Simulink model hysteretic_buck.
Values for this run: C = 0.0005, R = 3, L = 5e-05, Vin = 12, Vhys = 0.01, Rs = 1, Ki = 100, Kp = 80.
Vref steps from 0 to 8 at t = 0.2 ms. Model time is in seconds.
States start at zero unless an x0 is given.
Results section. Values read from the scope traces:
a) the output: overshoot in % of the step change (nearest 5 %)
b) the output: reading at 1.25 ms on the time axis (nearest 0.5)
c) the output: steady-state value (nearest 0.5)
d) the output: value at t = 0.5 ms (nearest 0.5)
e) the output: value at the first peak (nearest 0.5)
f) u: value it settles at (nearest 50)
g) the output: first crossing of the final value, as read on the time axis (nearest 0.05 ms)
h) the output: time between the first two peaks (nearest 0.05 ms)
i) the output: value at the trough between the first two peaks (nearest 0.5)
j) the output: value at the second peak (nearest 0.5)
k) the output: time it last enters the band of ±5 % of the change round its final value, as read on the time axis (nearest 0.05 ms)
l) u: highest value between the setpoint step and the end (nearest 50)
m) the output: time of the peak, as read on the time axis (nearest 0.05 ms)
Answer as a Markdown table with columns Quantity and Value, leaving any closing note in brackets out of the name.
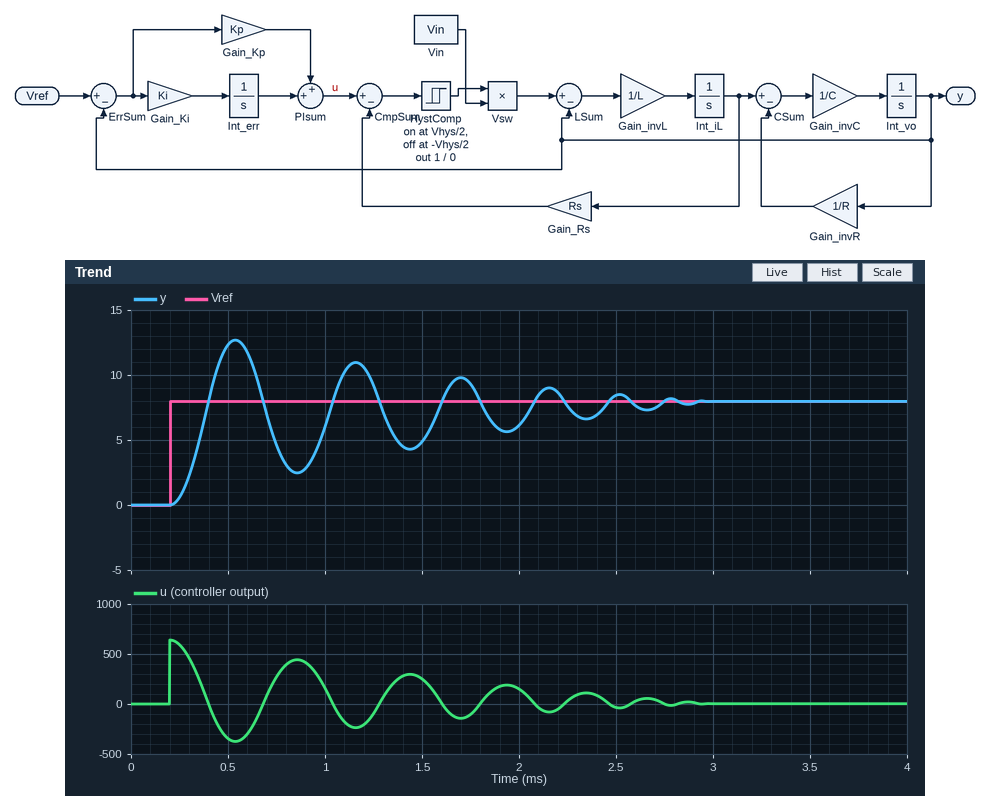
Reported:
| Quantity | Value |
|---|---|
| the output: overshoot in % of the step change | 60 % |
| the output: reading at 1.25 ms on the time axis | 9.0 |
| the output: steady-state value | 8.0 |
| the output: value at t = 0.5 ms | 12.5 |
| the output: value at the first peak | 12.5 |
| u: value it settles at | 0 |
| the output: first crossing of the final value, as read on the time axis | 0.40 ms |
| the output: time between the first two peaks | 0.60 ms |
| the output: value at the trough between the first two peaks | 2.5 |
| the output: value at the second peak | 11.0 |
| the output: time it last enters the band of ±5 % of the change round its final value, as read on the time axis | 2.70 ms |
| u: highest value between the setpoint step and the end | 650 |
| the output: time of the peak, as read on the time axis | 0.55 ms |
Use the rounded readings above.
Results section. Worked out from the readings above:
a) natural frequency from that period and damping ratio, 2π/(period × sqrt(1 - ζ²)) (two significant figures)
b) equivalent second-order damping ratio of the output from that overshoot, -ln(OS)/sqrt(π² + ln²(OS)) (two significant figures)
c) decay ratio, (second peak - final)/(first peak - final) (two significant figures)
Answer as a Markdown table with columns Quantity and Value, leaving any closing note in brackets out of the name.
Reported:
| Quantity | Value |
|---|---|
| natural frequency from that period and damping ratio, 2π/(period × sqrt(1 - ζ²)) | 11 rad/ms |
| equivalent second-order damping ratio of the output from that overshoot, -ln(OS)/sqrt(π² + ln²(OS)) | 0.16 |
| decay ratio, (second peak - final)/(first peak - final) | 0.67 |
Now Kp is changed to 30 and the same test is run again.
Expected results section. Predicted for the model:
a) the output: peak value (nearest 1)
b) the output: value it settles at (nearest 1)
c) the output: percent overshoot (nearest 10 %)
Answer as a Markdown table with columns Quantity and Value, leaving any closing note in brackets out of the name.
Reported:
| Quantity | Value |
|---|---|
| the output: peak value | 12 |
| the output: value it settles at | 8 |
| the output: percent overshoot | 50 % |
